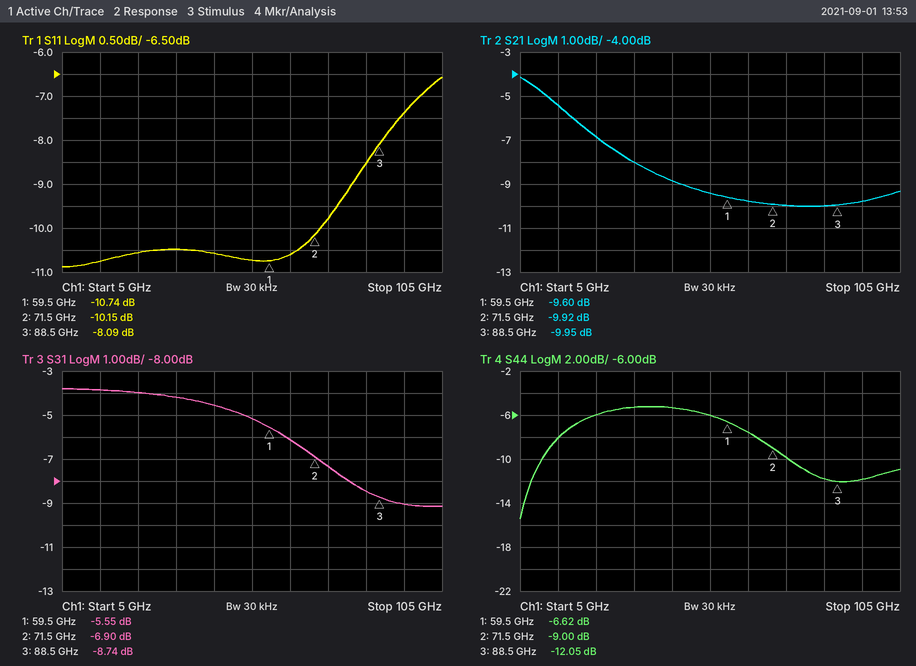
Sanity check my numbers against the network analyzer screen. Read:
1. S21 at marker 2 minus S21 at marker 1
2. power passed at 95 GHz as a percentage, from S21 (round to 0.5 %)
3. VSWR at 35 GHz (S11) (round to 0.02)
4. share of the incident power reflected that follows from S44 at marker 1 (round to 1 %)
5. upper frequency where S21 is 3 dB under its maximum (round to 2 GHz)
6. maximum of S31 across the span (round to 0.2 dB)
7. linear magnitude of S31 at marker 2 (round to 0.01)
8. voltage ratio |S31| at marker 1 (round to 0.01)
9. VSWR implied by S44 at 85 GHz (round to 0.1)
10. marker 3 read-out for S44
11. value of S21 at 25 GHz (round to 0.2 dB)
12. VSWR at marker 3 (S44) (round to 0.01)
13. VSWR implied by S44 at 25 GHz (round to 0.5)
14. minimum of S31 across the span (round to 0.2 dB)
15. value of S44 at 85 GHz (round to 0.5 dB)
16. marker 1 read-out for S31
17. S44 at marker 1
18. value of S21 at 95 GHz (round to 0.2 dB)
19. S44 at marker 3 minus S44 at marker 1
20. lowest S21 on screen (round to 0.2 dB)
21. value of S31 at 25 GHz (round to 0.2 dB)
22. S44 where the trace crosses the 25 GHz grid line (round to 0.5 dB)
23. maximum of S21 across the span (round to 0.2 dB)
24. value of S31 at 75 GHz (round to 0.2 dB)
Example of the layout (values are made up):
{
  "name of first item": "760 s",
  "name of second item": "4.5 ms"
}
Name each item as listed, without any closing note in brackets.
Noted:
{
  "S21 at marker 2 minus S21 at marker 1": "-0.32 dB",
  "power passed at 95 GHz as a percentage, from S21": "10.5 %",
  "VSWR at 35 GHz (S11)": "1.86",
  "share of the incident power reflected that follows from S44 at marker 1": "22 %",
  "upper frequency where S21 is 3 dB under its maximum": "28 GHz",
  "maximum of S31 across the span": "-3.8 dB",
  "linear magnitude of S31 at marker 2": "0.45",
  "voltage ratio |S31| at marker 1": "0.53",
  "VSWR implied by S44 at 85 GHz": "1.7",
  "marker 3 read-out for S44": "-12.05 dB",
  "value of S21 at 25 GHz": "-6.8 dB",
  "VSWR at marker 3 (S44)": "1.67",
  "VSWR implied by S44 at 25 GHz": "3.0",
  "minimum of S31 across the span": "-9.2 dB",
  "value of S44 at 85 GHz": "-12.0 dB",
  "marker 1 read-out for S31": "-5.55 dB",
  "S44 at marker 1": "-6.62 dB",
  "value of S21 at 95 GHz": "-9.8 dB",
  "S44 at marker 3 minus S44 at marker 1": "-5.43 dB",
  "lowest S21 on screen": "-10.0 dB",
  "value of S31 at 25 GHz": "-4.0 dB",
  "S44 where the trace crosses the 25 GHz grid line": "-6.0 dB",
  "maximum of S21 across the span": "-4.2 dB",
  "value of S31 at 75 GHz": "-7.4 dB"
}
